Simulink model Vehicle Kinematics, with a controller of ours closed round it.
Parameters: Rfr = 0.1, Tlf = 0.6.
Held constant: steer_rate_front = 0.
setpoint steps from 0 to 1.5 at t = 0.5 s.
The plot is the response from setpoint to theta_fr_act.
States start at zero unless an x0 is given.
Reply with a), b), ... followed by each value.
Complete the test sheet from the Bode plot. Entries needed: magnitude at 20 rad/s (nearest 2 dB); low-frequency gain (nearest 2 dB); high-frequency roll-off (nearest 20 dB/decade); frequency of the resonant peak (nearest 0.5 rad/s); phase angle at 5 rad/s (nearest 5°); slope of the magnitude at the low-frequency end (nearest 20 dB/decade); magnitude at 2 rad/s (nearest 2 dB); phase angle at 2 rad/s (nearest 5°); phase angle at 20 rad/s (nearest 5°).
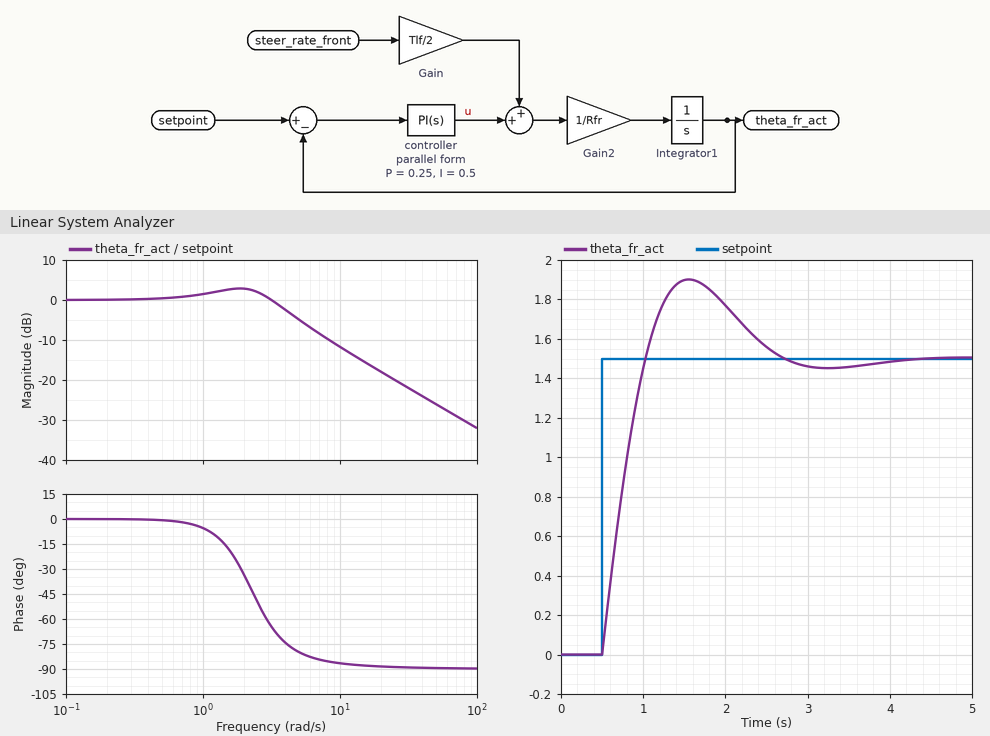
a) -18 dB
b) 0 dB
c) -20 dB/decade
d) 2.0 rad/s
e) -80°
f) 0 dB/decade
g) 2 dB
h) -35°
i) -90°
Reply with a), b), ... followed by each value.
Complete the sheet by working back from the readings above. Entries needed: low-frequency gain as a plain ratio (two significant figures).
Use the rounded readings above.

a) 1.0
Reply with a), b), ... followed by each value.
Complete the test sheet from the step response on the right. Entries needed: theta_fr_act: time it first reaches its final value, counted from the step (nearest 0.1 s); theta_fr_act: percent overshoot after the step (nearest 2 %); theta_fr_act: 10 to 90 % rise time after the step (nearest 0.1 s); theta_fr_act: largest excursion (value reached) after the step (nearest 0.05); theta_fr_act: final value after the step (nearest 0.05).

a) 0.5 s
b) 26 %
c) 0.4 s
d) 1.90
e) 1.50
